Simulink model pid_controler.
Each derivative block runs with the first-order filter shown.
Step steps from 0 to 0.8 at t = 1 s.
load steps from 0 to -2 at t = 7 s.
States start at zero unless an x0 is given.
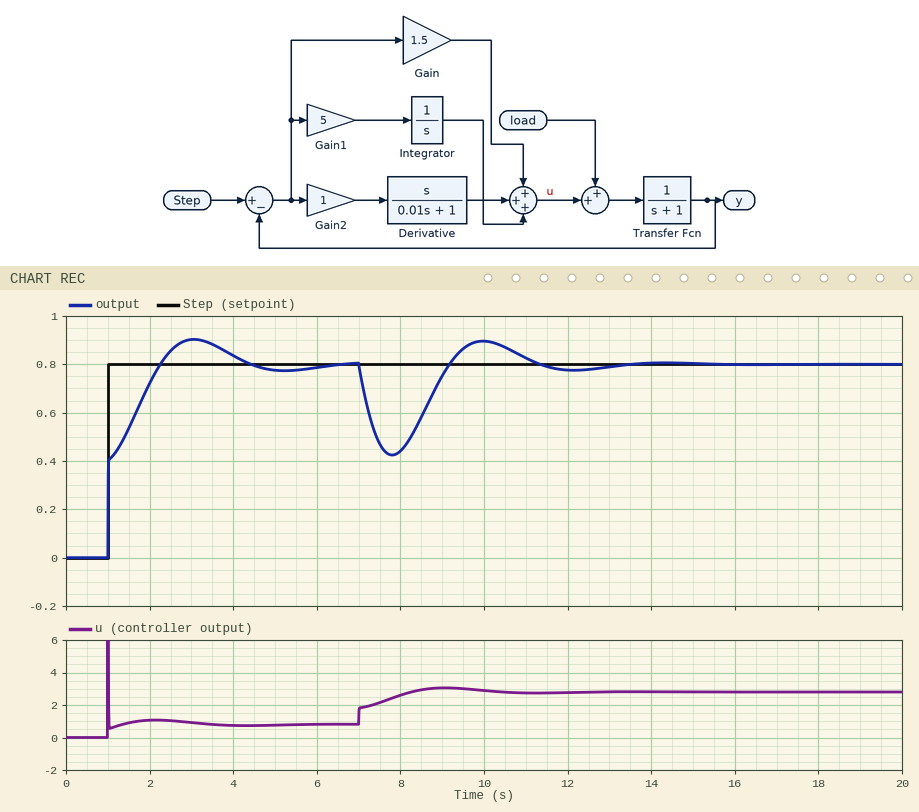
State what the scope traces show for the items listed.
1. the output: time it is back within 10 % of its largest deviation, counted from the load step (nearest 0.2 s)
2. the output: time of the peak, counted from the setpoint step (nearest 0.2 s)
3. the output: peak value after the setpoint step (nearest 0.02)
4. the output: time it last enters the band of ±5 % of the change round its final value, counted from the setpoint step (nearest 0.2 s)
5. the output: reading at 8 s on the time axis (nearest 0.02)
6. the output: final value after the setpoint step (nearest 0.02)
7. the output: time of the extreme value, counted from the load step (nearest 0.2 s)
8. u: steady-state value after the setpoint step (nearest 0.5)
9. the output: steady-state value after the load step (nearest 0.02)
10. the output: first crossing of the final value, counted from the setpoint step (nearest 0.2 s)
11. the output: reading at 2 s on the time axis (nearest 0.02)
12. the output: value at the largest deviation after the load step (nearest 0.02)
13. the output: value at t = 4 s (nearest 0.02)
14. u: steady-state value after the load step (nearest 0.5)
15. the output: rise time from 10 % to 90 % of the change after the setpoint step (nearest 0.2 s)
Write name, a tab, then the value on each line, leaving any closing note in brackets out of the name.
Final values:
the output: time it is back within 10 % of its largest deviation, counted from the load step	3.8 s
the output: time of the peak, counted from the setpoint step	2.0 s
the output: peak value after the setpoint step	0.90
the output: time it last enters the band of ±5 % of the change round its final value, counted from the setpoint step	3.0 s
the output: reading at 8 s on the time axis	0.44
the output: final value after the setpoint step	0.80
the output: time of the extreme value, counted from the load step	0.8 s
u: steady-state value after the setpoint step	1.0
the output: steady-state value after the load step	0.80
the output: first crossing of the final value, counted from the setpoint step	1.2 s
the output: reading at 2 s on the time axis	0.72
the output: value at the largest deviation after the load step	0.42
the output: value at t = 4 s	0.84
u: steady-state value after the load step	3.0
the output: rise time from 10 % to 90 % of the change after the setpoint step	1.0 s
